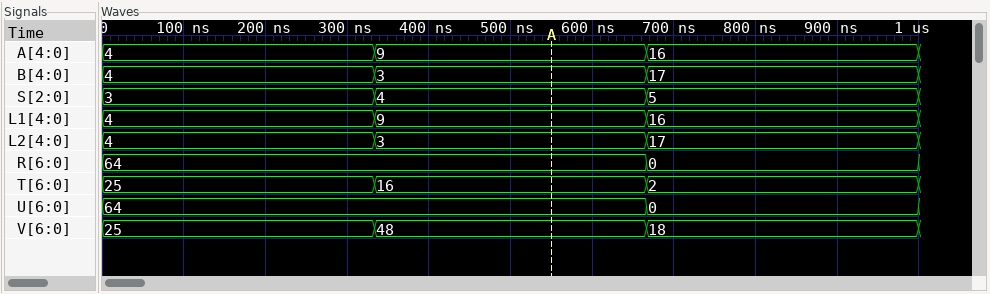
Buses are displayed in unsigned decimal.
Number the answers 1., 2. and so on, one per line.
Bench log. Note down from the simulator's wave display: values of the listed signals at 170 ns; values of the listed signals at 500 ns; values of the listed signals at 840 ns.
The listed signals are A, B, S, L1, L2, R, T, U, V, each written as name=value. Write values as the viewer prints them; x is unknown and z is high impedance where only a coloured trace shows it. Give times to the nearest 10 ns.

1. A=4, B=4, S=3, L1=4, L2=4, R=64, T=25, U=64, V=25
2. A=9, B=3, S=4, L1=9, L2=3, R=64, T=16, U=64, V=48
3. A=16, B=17, S=5, L1=16, L2=17, R=0, T=2, U=0, V=18
